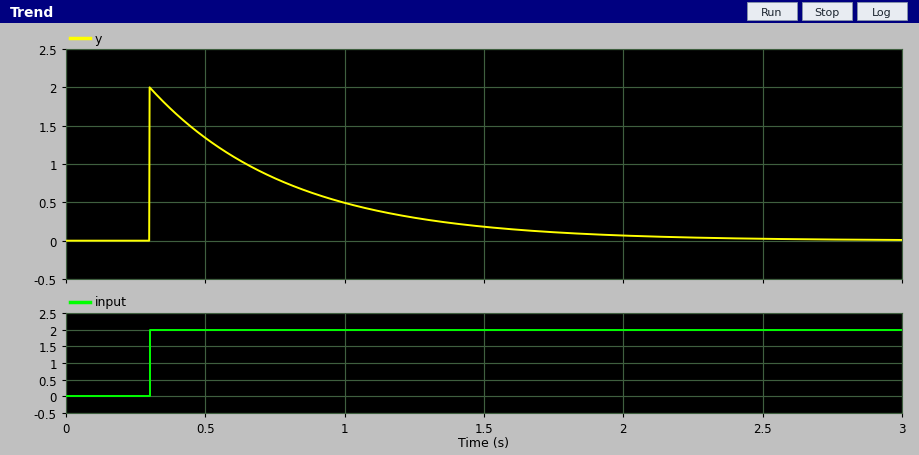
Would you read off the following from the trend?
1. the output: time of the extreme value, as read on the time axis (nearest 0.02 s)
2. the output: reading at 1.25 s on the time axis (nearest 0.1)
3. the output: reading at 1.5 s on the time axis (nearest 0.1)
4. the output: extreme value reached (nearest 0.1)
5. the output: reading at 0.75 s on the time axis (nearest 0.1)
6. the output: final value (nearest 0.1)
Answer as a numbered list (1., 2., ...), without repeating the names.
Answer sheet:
1. 0.30 s
2. 0.3
3. 0.2
4. 2.0
5. 0.8
6. 0.0
